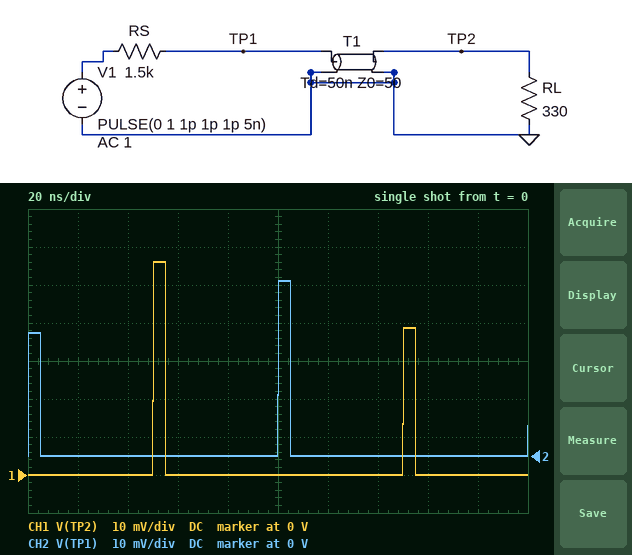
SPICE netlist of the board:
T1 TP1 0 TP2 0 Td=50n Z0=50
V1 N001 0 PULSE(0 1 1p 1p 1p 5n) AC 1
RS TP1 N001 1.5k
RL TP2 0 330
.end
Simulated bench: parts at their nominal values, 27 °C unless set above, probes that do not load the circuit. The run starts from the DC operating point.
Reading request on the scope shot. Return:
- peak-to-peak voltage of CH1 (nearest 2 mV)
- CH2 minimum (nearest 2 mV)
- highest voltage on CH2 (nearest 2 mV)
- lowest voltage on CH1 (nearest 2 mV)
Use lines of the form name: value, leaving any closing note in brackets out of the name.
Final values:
peak-to-peak voltage of CH1: 56 mV
CH2 minimum: 0 V
highest voltage on CH2: 46 mV
lowest voltage on CH1: 0 V
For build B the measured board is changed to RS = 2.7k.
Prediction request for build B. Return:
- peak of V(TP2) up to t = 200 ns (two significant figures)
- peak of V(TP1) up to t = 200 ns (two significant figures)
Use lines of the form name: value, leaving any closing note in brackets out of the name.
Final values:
peak of V(TP2) up to t = 200 ns: 32 mV
peak of V(TP1) up to t = 200 ns: 26 mV
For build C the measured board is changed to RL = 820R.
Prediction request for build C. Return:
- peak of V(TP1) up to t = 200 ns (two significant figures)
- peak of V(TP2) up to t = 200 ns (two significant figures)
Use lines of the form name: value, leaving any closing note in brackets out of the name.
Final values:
peak of V(TP1) up to t = 200 ns: 55 mV
peak of V(TP2) up to t = 200 ns: 61 mV
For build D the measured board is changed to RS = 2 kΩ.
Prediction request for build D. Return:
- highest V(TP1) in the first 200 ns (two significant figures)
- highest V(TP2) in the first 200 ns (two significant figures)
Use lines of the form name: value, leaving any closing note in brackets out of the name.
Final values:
highest V(TP1) in the first 200 ns: 35 mV
highest V(TP2) in the first 200 ns: 42 mV
